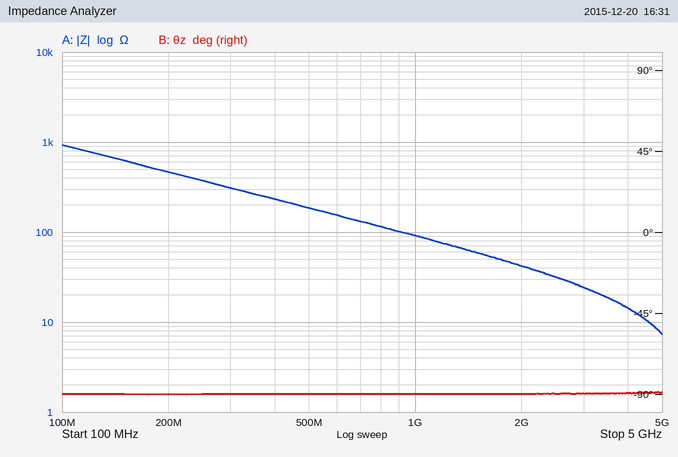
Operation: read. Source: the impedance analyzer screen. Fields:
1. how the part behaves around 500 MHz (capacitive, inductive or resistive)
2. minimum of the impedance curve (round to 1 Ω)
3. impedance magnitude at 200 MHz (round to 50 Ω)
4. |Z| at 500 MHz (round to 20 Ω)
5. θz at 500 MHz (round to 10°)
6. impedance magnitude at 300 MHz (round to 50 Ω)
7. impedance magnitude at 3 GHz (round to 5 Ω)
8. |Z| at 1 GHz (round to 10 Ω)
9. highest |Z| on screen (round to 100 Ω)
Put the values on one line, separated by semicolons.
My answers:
capacitive; 7 Ω; 450 Ω; 180 Ω; -90°; 300 Ω; 25 Ω; 90 Ω; 900 Ω
